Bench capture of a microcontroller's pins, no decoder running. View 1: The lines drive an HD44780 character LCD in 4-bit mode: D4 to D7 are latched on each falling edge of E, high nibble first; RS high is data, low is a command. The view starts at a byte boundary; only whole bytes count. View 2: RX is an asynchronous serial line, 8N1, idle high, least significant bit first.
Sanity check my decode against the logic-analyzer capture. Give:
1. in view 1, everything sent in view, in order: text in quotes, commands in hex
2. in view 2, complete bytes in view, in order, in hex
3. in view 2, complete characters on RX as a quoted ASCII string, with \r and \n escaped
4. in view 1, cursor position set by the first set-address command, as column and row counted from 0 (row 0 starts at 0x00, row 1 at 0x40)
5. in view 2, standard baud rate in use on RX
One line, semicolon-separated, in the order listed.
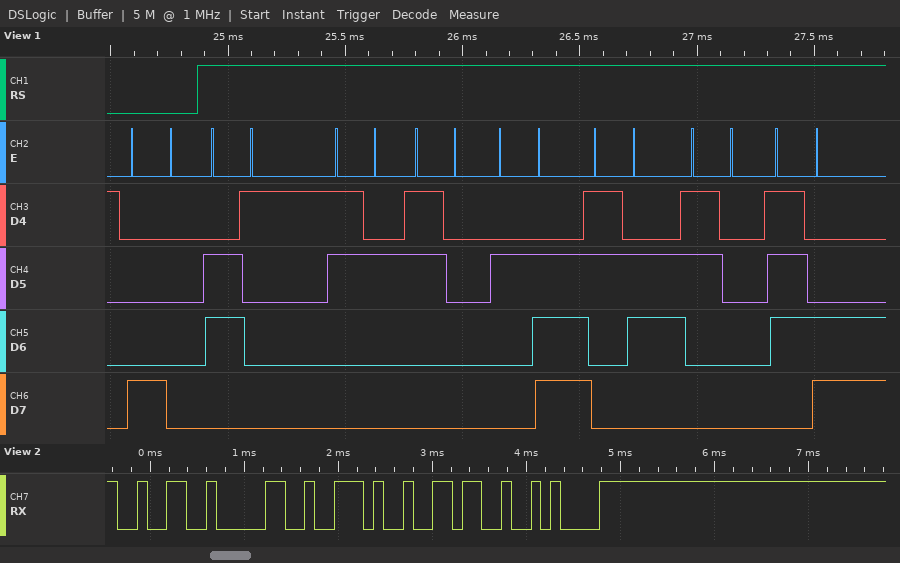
0x80 "a20.60|"; 32 30 2E 36 0A; "20.6\n"; column 0, row 0; 9600 baud
